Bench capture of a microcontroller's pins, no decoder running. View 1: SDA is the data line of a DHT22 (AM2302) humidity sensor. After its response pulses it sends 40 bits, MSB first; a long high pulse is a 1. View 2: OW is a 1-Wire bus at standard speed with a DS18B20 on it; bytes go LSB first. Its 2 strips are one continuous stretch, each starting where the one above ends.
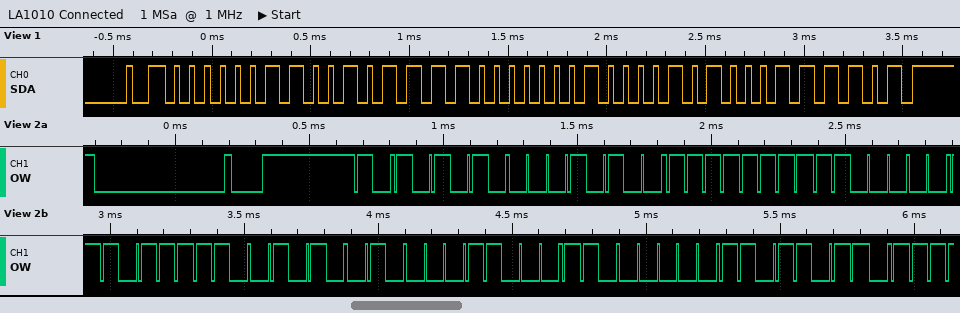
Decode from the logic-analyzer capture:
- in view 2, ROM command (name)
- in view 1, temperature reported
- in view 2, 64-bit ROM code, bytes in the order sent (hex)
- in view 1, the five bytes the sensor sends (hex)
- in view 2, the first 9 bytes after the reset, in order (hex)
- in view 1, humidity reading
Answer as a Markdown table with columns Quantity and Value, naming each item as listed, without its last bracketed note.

| Quantity | Value |
|---|---|
| in view 2, ROM command | Match ROM |
| in view 1, temperature reported | 26.6 °C |
| in view 2, 64-bit ROM code, bytes in the order sent | 28 FF 83 7D 4A 18 03 DB |
| in view 1, the five bytes the sensor sends | 03 2F 01 0A 3D |
| in view 2, the first 9 bytes after the reset, in order | 55 28 FF 83 7D 4A 18 03 DB |
| in view 1, humidity reading | 81.5 % |
